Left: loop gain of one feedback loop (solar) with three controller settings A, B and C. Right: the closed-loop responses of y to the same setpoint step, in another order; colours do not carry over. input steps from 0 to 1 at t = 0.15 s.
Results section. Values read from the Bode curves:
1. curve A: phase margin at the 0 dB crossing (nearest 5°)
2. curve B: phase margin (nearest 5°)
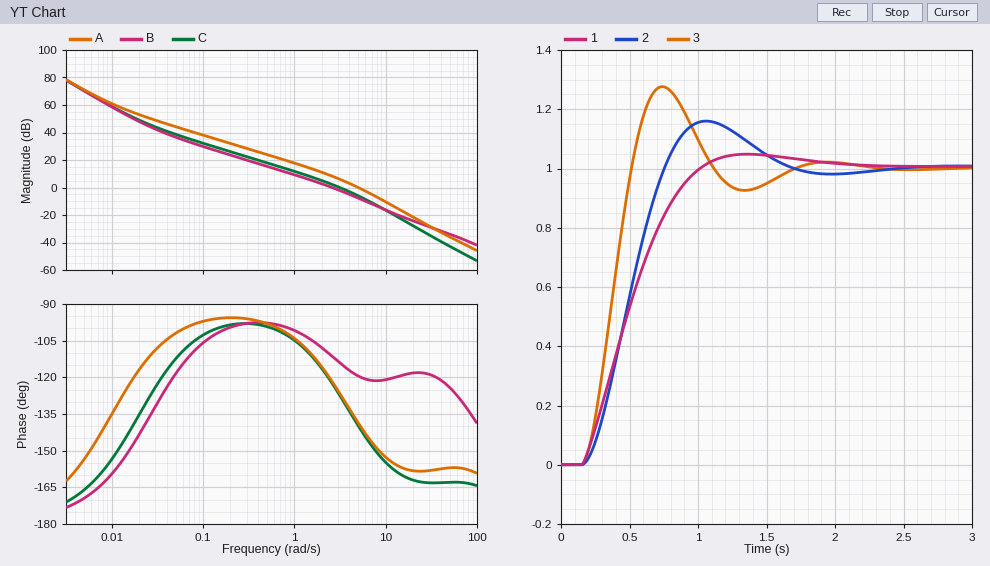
40°
70°
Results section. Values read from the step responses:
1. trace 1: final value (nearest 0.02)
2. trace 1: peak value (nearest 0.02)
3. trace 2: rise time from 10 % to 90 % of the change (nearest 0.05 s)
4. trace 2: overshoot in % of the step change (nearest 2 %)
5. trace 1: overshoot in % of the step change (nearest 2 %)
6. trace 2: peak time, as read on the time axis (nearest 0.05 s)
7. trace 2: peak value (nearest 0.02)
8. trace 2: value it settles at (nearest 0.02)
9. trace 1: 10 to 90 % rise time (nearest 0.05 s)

1.00
1.04
0.40 s
16 %
4 %
1.05 s
1.16
1.00
0.60 s
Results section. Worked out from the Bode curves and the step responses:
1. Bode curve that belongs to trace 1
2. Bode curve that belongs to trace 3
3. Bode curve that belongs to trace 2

B
A
C
